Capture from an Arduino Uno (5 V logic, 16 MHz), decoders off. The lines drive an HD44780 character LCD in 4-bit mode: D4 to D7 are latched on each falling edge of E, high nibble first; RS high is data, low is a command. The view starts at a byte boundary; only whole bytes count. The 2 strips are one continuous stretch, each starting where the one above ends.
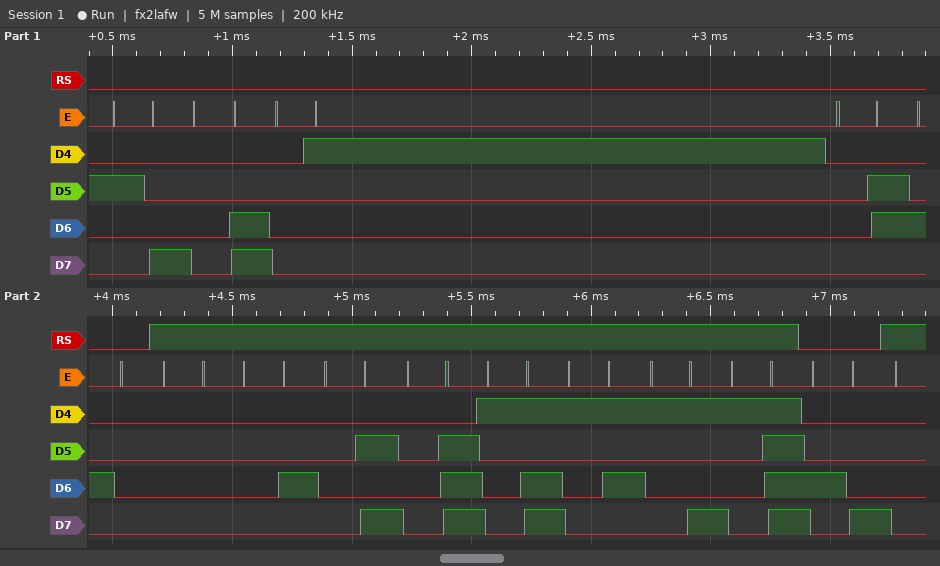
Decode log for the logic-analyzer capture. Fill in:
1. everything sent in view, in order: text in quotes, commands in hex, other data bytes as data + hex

0x28 0x0C 0x01 0x06 0x40 data 00 04 0A 0E 1D 15 19 1F 0x48
